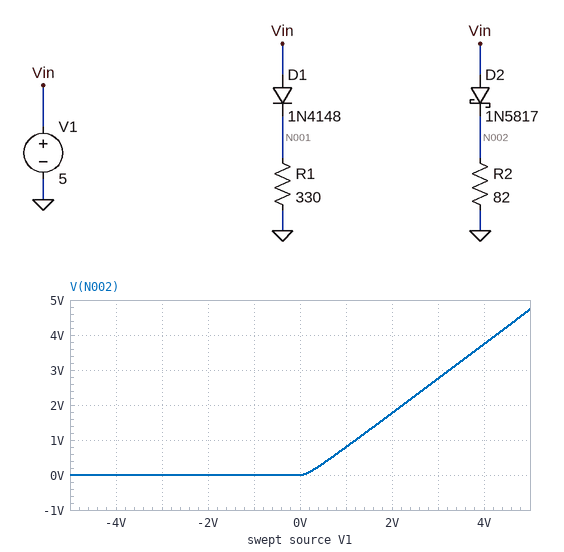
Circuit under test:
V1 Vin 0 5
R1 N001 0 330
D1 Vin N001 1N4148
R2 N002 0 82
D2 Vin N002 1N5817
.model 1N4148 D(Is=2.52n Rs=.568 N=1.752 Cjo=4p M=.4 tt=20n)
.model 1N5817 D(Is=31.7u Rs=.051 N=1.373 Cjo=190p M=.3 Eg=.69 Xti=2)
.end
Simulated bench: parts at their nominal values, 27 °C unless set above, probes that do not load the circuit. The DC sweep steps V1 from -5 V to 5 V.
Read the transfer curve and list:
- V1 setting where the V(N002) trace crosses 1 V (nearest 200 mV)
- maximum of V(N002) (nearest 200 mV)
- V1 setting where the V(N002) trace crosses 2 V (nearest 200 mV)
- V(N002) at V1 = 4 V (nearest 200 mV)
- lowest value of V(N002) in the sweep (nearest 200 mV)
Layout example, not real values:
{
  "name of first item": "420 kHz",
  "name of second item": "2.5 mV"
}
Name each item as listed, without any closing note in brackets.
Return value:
{
  "V1 setting where the V(N002) trace crosses 1 V": "1.2 V",
  "maximum of V(N002)": "4.8 V",
  "V1 setting where the V(N002) trace crosses 2 V": "2.2 V",
  "V(N002) at V1 = 4 V": "3.8 V",
  "lowest value of V(N002) in the sweep": "0 V"
}
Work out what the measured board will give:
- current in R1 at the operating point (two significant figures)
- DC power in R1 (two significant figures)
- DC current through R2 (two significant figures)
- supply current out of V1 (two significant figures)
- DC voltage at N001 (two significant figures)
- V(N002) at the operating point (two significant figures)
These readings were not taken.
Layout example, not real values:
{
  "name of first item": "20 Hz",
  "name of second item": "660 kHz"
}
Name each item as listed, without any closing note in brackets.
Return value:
{
  "current in R1 at the operating point": "13 mA",
  "DC power in R1": "56 mW",
  "DC current through R2": "58 mA",
  "supply current out of V1": "71 mA",
  "DC voltage at N001": "4.3 V",
  "V(N002) at the operating point": "4.7 V"
}
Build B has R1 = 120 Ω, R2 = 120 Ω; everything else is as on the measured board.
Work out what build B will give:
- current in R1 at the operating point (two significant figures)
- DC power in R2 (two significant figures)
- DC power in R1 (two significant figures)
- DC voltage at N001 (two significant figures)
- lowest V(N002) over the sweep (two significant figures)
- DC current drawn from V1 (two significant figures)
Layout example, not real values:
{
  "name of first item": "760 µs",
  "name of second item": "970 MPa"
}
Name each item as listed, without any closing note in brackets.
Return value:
{
  "current in R1 at the operating point": "35 mA",
  "DC power in R2": "190 mW",
  "DC power in R1": "150 mW",
  "DC voltage at N001": "4.2 V",
  "lowest V(N002) over the sweep": "-3.8 mV",
  "DC current drawn from V1": "75 mA"
}
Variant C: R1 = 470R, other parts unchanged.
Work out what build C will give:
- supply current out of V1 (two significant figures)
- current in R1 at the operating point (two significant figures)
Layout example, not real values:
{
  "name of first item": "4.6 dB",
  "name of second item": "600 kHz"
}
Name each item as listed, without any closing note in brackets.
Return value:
{
  "supply current out of V1": "67 mA",
  "current in R1 at the operating point": "9.2 mA"
}
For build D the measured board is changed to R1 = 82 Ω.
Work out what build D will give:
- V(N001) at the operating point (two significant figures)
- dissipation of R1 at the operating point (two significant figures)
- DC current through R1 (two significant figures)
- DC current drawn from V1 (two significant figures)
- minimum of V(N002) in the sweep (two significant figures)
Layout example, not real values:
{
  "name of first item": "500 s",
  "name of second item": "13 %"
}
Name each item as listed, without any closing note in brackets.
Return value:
{
  "V(N001) at the operating point": "4.2 V",
  "dissipation of R1 at the operating point": "220 mW",
  "DC current through R1": "51 mA",
  "DC current drawn from V1": "110 mA",
  "minimum of V(N002) in the sweep": "-2.6 mV"
}
